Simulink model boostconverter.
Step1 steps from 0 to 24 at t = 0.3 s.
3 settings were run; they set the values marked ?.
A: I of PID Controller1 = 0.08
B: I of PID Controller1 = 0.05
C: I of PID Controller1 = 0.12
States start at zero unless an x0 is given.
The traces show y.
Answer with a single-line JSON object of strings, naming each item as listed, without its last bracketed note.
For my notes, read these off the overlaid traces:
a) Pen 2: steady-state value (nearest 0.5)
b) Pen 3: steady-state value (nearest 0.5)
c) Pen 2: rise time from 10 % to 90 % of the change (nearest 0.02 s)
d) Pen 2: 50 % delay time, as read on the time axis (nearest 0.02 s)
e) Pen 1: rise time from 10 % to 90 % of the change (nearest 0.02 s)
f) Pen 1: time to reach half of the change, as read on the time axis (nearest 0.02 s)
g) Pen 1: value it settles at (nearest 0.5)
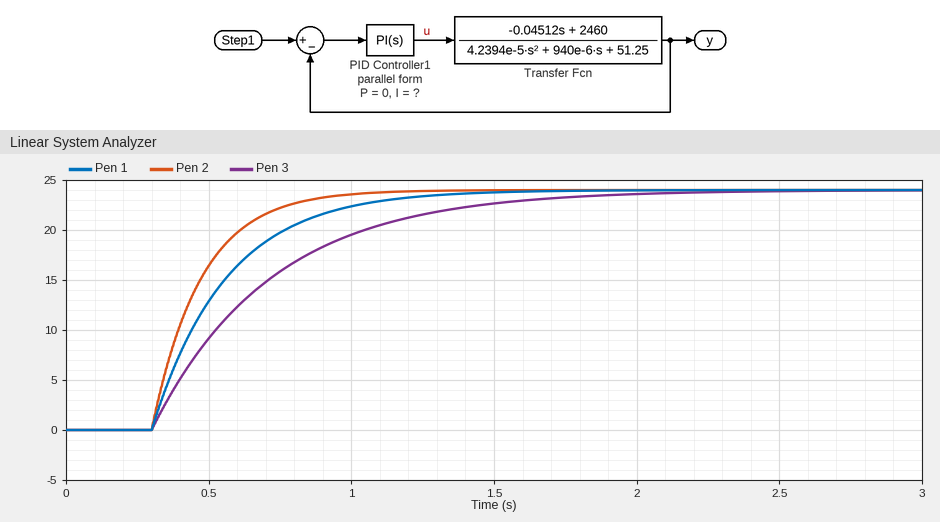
{"Pen 2: steady-state value": "24.0", "Pen 3: steady-state value": "24.0", "Pen 2: rise time from 10 % to 90 % of the change": "0.38 s", "Pen 2: 50 % delay time, as read on the time axis": "0.42 s", "Pen 1: rise time from 10 % to 90 % of the change": "0.58 s", "Pen 1: time to reach half of the change, as read on the time axis": "0.48 s", "Pen 1: value it settles at": "24.0"}
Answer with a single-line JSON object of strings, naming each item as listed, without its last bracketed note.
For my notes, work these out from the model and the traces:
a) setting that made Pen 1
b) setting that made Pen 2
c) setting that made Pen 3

{"setting that made Pen 1": "A", "setting that made Pen 2": "C", "setting that made Pen 3": "B"}
